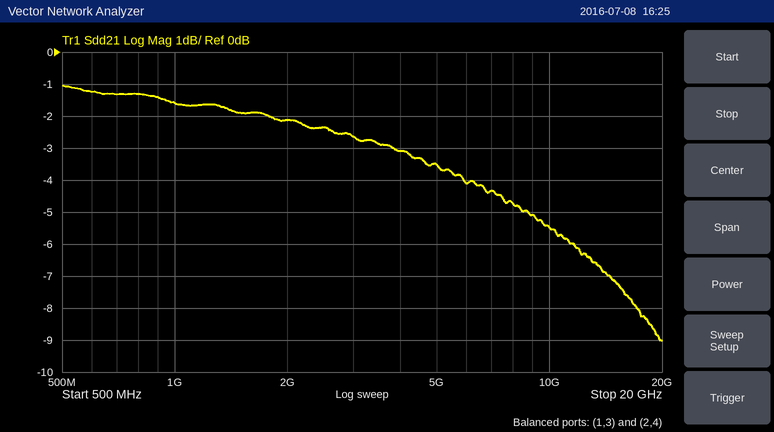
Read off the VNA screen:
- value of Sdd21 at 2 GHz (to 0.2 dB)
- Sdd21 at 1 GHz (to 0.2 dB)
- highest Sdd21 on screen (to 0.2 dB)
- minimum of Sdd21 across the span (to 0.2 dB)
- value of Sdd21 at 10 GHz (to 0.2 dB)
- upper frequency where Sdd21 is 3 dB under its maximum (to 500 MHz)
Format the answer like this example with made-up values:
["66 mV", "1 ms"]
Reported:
["-2.2 dB", "-1.6 dB", "-1.0 dB", "-9.0 dB", "-5.4 dB", "6.0 GHz"]
